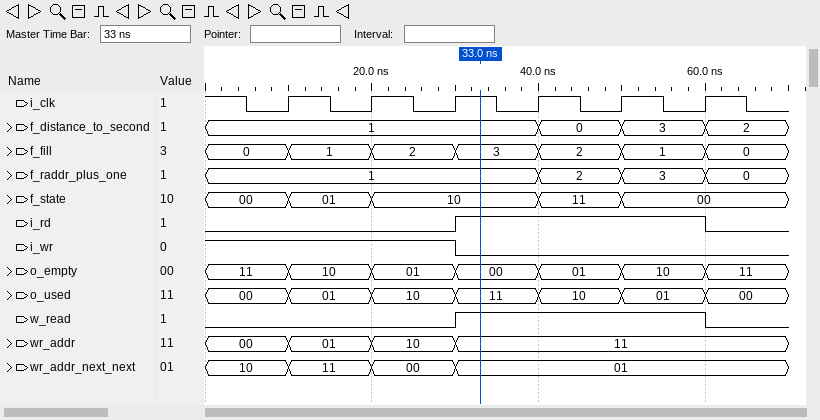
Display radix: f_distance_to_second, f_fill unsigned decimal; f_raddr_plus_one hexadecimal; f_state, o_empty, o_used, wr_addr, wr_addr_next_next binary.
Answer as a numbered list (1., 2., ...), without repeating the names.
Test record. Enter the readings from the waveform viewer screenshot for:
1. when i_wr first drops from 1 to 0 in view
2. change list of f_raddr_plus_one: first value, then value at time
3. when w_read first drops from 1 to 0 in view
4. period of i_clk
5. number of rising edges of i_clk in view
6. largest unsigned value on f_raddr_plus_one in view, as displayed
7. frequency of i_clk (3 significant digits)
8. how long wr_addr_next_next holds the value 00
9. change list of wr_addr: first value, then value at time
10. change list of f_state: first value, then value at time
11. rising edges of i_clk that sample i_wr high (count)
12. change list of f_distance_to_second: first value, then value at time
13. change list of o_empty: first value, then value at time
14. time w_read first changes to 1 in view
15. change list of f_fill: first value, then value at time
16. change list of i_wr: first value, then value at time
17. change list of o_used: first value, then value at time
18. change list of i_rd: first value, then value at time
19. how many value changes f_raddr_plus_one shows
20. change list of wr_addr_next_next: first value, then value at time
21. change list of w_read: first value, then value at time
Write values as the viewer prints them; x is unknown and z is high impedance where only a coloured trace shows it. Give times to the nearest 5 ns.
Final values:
1. 30 ns
2. 1, 2 at 40 ns, 3 at 50 ns, 0 at 60 ns
3. 60 ns
4. 10 ns
5. 6
6. 3
7. 100 MHz
8. 10 ns
9. 00, 01 at 10 ns, 10 at 20 ns, 11 at 30 ns
10. 00, 01 at 10 ns, 10 at 20 ns, 11 at 40 ns, 00 at 50 ns
11. 3
12. 1, 0 at 40 ns, 3 at 50 ns, 2 at 60 ns
13. 11, 10 at 10 ns, 01 at 20 ns, 00 at 30 ns, 01 at 40 ns, 10 at 50 ns, 11 at 60 ns
14. 30 ns
15. 0, 1 at 10 ns, 2 at 20 ns, 3 at 30 ns, 2 at 40 ns, 1 at 50 ns, 0 at 60 ns
16. 1, 0 at 30 ns
17. 00, 01 at 10 ns, 10 at 20 ns, 11 at 30 ns, 10 at 40 ns, 01 at 50 ns, 00 at 60 ns
18. 0, 1 at 30 ns, 0 at 60 ns
19. 3
20. 10, 11 at 10 ns, 00 at 20 ns, 01 at 30 ns
21. 0, 1 at 30 ns, 0 at 60 ns
